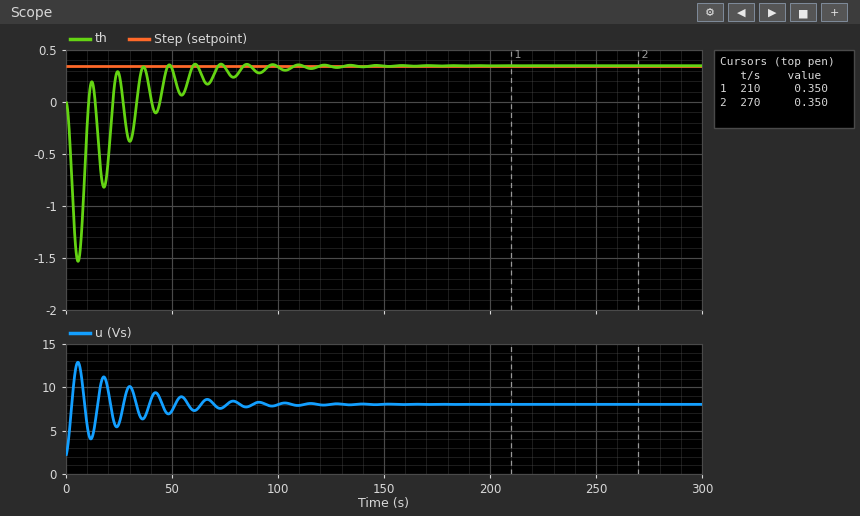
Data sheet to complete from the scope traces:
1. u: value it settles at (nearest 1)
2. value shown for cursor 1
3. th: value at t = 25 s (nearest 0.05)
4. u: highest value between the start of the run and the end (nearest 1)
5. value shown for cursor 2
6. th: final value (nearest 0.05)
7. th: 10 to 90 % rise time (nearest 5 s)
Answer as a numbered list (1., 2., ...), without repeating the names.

1. 8
2. 0.350
3. 0.25
4. 13
5. 0.350
6. 0.35
7. 25 s
